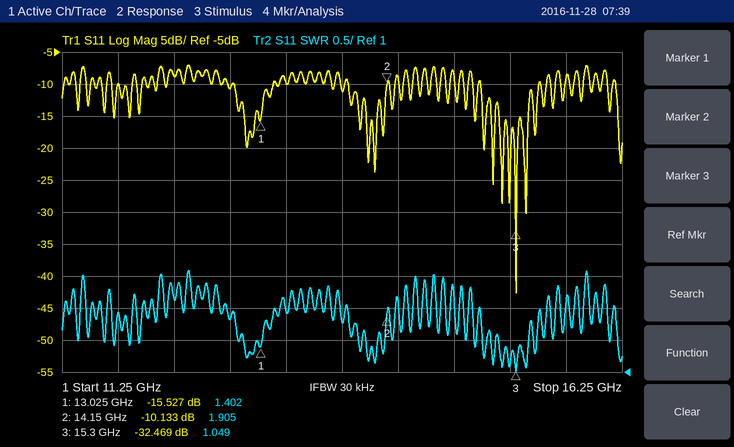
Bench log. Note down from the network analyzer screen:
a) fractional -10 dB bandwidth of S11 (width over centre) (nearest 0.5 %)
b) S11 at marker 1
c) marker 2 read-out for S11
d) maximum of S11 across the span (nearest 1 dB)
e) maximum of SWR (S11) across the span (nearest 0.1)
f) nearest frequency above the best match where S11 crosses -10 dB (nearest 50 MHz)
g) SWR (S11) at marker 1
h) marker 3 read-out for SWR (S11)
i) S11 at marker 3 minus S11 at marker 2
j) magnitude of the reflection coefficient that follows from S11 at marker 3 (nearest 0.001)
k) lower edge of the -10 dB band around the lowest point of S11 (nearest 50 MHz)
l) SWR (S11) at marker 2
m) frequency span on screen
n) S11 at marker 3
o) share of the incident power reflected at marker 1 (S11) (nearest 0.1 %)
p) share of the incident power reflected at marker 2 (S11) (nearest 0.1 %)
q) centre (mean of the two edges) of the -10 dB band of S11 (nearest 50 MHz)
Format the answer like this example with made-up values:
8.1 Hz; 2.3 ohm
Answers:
3.5 %; -15.527 dB; -10.133 dB; -7 dB; 2.6; 15.50 GHz; 1.402; 1.049; -22.336 dB; 0.024; 15.00 GHz; 1.905; 5 GHz; -32.469 dB; 2.8 %; 9.7 %; 15.25 GHz
